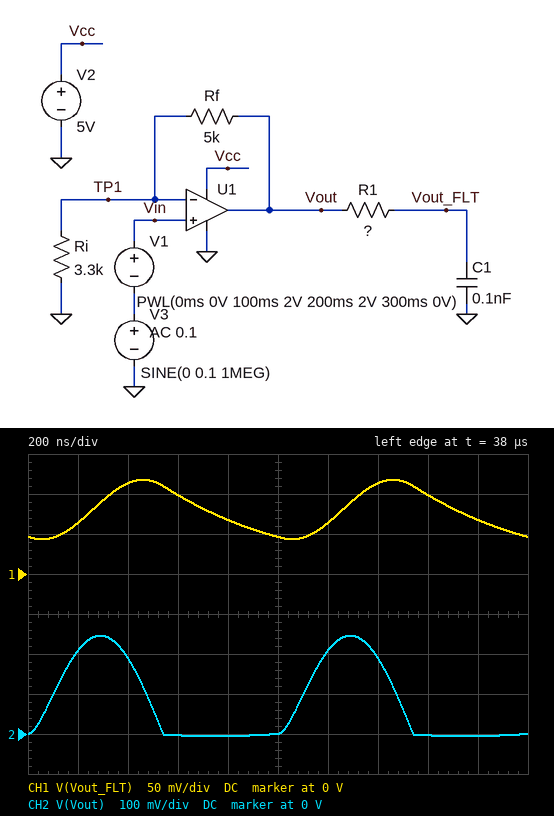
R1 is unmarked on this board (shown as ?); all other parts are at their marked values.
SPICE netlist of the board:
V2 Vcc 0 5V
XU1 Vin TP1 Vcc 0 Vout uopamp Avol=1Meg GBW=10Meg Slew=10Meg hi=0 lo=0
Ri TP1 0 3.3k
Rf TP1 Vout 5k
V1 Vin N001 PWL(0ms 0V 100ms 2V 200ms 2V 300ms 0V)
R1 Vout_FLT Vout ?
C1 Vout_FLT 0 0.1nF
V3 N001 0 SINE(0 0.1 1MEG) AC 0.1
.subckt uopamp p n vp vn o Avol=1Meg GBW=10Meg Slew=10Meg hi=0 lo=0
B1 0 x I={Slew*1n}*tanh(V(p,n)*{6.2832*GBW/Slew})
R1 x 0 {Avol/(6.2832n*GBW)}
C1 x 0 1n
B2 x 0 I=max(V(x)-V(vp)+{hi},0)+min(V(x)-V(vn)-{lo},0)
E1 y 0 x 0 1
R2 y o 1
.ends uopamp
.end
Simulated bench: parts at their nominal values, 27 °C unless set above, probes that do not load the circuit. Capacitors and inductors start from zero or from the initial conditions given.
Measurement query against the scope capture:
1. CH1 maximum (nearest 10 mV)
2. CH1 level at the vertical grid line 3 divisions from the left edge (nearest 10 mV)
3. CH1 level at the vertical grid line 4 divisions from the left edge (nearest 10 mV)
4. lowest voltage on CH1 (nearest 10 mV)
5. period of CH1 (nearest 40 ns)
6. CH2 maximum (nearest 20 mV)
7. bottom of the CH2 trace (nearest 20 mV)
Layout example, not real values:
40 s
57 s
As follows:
120 mV
100 mV
70 mV
40 mV
1.00 µs
240 mV
0 V
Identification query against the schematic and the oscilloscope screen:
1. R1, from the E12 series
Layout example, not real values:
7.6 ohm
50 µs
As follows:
5.6 kΩ
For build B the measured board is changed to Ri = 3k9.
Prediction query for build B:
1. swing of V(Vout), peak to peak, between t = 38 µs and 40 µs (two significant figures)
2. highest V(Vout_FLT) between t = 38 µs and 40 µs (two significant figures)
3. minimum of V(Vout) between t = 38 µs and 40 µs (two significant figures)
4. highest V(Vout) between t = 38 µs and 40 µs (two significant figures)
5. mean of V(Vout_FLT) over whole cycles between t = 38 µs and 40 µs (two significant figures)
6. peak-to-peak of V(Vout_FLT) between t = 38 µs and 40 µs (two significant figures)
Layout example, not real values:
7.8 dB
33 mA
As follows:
230 mV
110 mV
-5.4 mV
220 mV
71 mV
68 mV
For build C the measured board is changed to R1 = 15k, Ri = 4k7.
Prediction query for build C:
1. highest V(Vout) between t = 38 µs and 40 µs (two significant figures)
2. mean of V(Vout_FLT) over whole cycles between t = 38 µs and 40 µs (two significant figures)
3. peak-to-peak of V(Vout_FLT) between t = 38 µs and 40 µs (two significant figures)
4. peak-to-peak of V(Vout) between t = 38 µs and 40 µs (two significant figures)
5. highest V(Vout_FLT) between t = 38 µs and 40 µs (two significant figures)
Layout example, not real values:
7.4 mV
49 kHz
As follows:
200 mV
64 mV
24 mV
210 mV
76 mV
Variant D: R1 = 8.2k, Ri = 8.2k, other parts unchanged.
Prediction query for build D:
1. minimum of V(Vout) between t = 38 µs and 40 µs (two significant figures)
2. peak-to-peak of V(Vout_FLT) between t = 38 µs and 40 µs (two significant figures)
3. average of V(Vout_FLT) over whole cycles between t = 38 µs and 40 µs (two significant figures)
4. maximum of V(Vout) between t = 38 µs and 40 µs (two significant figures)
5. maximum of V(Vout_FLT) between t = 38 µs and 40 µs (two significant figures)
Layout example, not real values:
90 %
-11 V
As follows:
-5.4 mV
34 mV
50 mV
160 mV
68 mV
